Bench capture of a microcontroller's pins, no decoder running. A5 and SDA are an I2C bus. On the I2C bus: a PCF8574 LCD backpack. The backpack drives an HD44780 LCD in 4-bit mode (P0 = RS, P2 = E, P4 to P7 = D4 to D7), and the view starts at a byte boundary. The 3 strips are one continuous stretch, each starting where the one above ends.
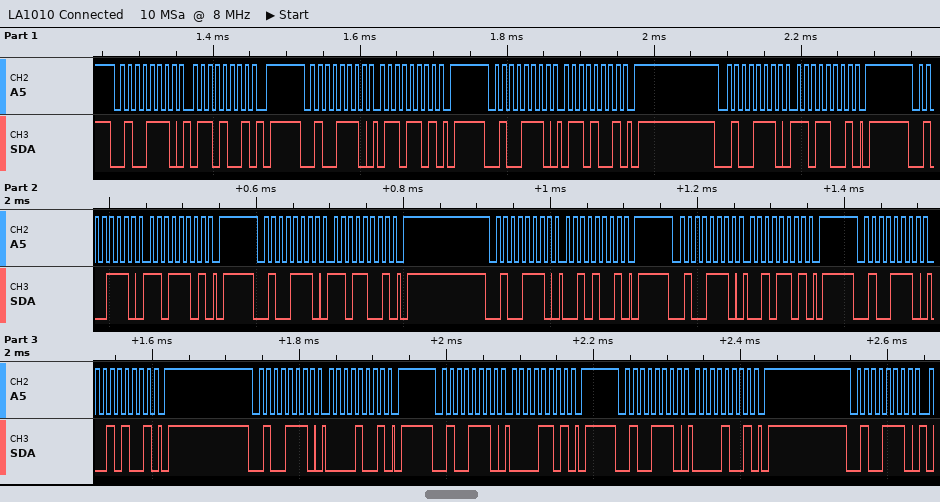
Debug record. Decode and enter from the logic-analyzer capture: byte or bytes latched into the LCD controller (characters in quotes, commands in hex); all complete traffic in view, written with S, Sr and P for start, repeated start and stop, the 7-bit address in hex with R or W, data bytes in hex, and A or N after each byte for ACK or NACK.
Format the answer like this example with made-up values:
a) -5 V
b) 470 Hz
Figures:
a) 'm' ' '
b) S 27W A 69 A P S 27W A 6D A P S 27W A 69 A P S 27W A D9 A P S 27W A DD A P S 27W A D9 A P S 27W A 29 A P S 27W A 2D A P S 27W A 29 A P S 27W A 09 A P S 27W A 0D A P S 27W A 09 A P S 27W A
